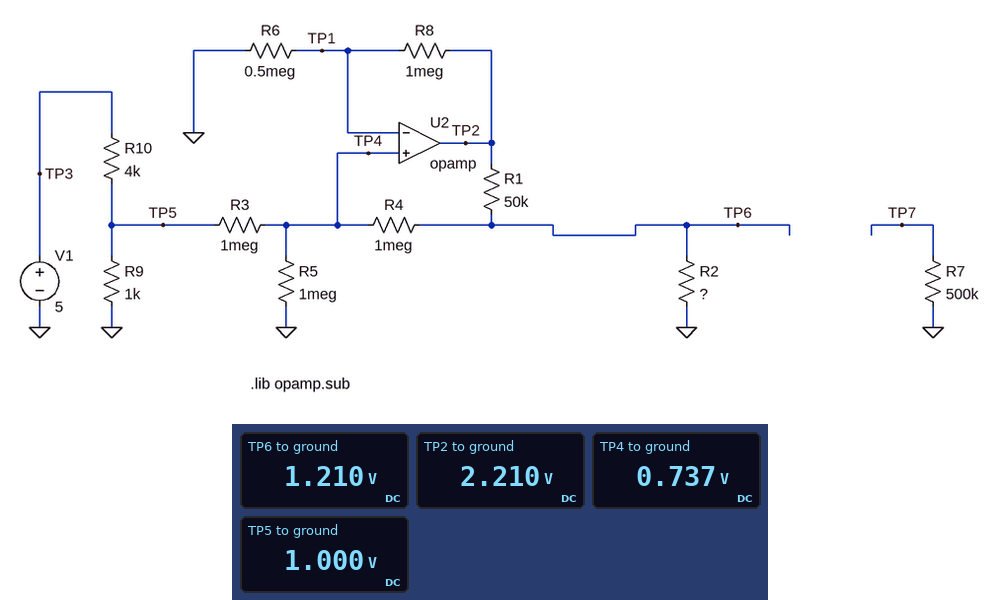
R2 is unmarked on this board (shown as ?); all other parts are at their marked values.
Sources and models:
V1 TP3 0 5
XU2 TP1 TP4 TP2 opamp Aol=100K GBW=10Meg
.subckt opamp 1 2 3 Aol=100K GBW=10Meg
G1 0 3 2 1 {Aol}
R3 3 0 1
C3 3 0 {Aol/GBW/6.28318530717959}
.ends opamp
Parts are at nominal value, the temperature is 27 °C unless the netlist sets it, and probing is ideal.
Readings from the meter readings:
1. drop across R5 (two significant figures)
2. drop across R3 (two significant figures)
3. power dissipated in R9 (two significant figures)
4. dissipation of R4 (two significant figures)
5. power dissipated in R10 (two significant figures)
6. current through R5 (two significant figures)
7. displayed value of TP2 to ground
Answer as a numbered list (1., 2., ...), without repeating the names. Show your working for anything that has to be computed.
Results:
1. 737 mV = 740 mV
2. 1 V - 737 mV = 260 mV
3. (1 V)^2 / 1 kΩ = 1.0 mW
4. (1.21 V - 737 mV)^2 / 1 MΩ = 220 nW
5. (5 V - 1 V)^2 / 4 kΩ = 4.0 mW
6. (737 mV) / 1 MΩ = 740 nA
7. 2.210 V
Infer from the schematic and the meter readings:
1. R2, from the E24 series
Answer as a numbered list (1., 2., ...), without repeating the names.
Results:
1. 62 kΩ
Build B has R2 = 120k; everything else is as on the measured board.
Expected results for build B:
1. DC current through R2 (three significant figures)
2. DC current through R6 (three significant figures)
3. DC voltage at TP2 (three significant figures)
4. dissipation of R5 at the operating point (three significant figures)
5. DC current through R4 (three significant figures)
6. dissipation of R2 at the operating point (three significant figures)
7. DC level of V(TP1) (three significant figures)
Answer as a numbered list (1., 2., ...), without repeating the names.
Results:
1. 18.8 µA
2. 2.17 µA
3. 3.26 V
4. 1.18 µW
5. 1.17 µA
6. 42.5 µW
7. 1.09 V
